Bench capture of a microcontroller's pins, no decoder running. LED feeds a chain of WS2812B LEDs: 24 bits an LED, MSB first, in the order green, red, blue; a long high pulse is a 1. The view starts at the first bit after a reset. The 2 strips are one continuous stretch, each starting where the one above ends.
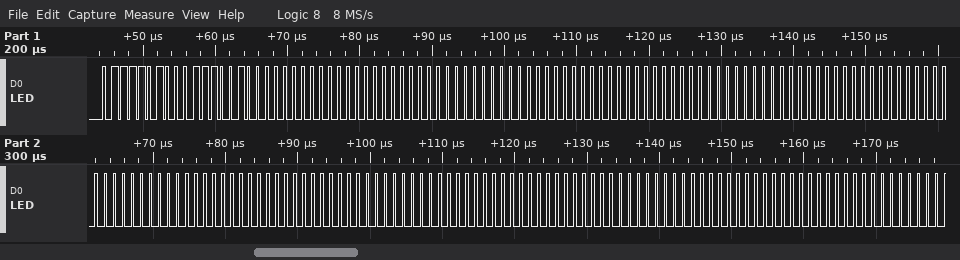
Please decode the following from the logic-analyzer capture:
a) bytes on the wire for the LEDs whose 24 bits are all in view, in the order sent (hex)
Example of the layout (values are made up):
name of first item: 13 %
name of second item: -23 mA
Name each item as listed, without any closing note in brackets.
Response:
bytes on the wire for the LEDs whose 24 bits are all in view, in the order sent: 7A 39 00 00 00 00 00 00 00 00 00 00 00 00 00 00 00 00 00 00 00
